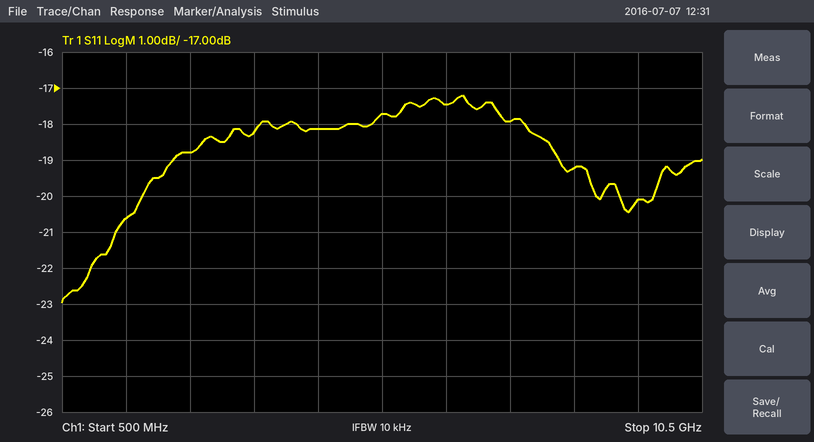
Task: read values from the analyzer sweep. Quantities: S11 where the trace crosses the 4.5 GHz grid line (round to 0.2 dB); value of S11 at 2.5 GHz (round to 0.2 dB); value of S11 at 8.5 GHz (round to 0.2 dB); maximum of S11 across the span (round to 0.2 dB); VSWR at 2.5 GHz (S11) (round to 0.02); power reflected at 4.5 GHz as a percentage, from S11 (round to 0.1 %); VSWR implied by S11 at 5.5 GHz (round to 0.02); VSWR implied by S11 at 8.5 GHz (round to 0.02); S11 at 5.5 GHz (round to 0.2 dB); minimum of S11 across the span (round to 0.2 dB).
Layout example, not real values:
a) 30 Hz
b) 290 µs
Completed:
a) -18.2 dB
b) -18.8 dB
c) -19.2 dB
d) -17.2 dB
e) 1.26
f) 1.5 %
g) 1.30
h) 1.24
i) -17.8 dB
j) -23.0 dB
